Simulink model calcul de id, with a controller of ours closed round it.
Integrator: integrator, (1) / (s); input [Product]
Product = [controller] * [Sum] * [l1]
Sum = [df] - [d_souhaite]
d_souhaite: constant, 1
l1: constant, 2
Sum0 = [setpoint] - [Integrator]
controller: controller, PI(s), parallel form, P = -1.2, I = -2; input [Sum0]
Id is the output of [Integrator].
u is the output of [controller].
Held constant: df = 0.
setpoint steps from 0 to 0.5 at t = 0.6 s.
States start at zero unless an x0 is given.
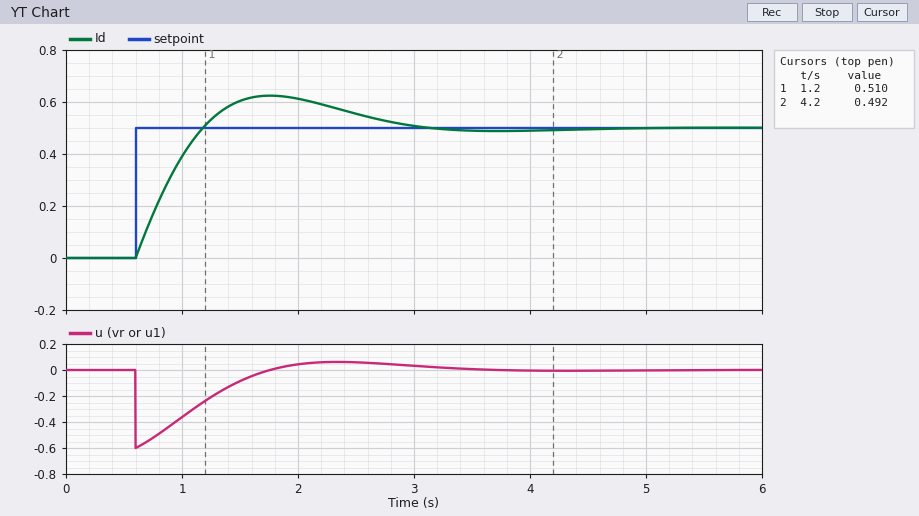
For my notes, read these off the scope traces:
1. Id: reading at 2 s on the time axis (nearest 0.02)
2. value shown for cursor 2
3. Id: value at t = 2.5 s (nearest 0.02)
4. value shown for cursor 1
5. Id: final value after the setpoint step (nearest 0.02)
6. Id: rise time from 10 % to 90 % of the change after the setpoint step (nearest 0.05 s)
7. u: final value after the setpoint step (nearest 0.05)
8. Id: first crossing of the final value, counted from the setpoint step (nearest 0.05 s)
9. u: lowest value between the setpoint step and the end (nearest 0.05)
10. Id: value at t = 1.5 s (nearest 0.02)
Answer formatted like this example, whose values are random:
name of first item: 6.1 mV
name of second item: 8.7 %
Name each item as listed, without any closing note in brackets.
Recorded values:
Id: reading at 2 s on the time axis: 0.62
value shown for cursor 2: 0.492
Id: value at t = 2.5 s: 0.56
value shown for cursor 1: 0.510
Id: final value after the setpoint step: 0.50
Id: rise time from 10 % to 90 % of the change after the setpoint step: 0.45 s
u: final value after the setpoint step: 0.00
Id: first crossing of the final value, counted from the setpoint step: 0.60 s
u: lowest value between the setpoint step and the end: -0.60
Id: value at t = 1.5 s: 0.60
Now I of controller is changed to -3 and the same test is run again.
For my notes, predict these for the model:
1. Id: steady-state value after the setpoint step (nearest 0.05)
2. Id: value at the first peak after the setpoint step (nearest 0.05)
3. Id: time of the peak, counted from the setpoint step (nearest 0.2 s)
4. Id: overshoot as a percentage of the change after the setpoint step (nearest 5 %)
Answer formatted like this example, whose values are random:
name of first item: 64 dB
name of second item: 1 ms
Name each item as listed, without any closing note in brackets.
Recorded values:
Id: steady-state value after the setpoint step: 0.50
Id: value at the first peak after the setpoint step: 0.65
Id: time of the peak, counted from the setpoint step: 1.0 s
Id: overshoot as a percentage of the change after the setpoint step: 30 %
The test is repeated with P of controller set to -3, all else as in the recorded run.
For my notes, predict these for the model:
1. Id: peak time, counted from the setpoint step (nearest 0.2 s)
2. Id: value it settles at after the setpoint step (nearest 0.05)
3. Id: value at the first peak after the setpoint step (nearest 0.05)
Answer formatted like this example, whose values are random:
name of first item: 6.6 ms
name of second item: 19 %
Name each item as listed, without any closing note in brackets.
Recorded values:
Id: peak time, counted from the setpoint step: 0.8 s
Id: value it settles at after the setpoint step: 0.50
Id: value at the first peak after the setpoint step: 0.55
